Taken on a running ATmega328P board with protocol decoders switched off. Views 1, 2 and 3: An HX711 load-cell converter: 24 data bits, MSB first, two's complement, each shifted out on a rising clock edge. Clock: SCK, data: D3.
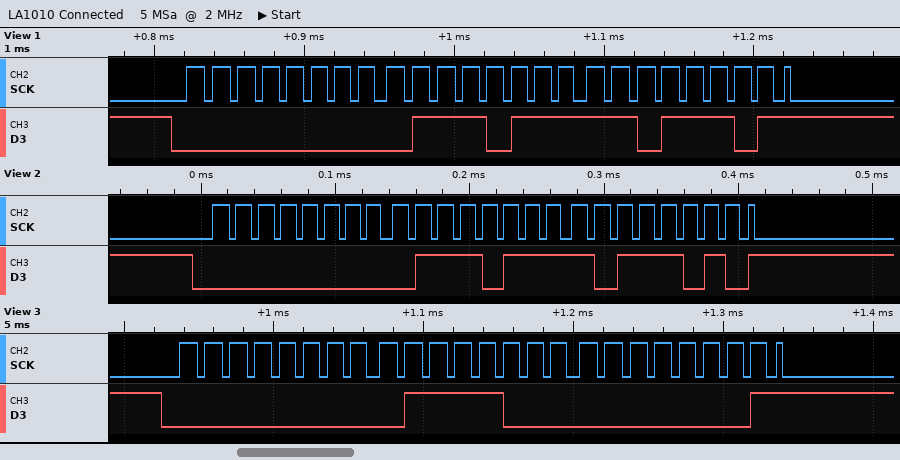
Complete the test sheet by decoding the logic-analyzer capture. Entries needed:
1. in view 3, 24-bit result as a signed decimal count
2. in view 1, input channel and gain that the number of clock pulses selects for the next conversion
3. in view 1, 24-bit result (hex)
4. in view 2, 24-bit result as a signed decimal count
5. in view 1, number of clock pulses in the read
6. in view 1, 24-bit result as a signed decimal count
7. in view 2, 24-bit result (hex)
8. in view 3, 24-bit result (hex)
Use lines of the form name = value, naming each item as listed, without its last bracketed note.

in view 3, 24-bit result as a signed decimal count = 30721
in view 1, input channel and gain that the number of clock pulses selects for the next conversion = channel A, gain 128
in view 1, 24-bit result = 0x0077DD
in view 2, 24-bit result as a signed decimal count = 30650
in view 1, number of clock pulses in the read = 25
in view 1, 24-bit result as a signed decimal count = 30685
in view 2, 24-bit result = 0x0077BA
in view 3, 24-bit result = 0x007801
